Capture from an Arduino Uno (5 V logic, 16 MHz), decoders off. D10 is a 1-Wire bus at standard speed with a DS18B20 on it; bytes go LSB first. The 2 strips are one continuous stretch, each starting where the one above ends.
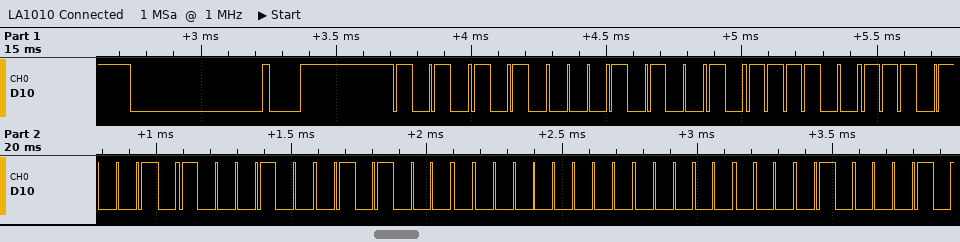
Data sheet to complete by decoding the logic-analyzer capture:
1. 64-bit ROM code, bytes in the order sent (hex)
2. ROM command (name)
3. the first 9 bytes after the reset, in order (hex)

28 3D 97 22 0A 00 00 42
Match ROM
55 28 3D 97 22 0A 00 00 42
